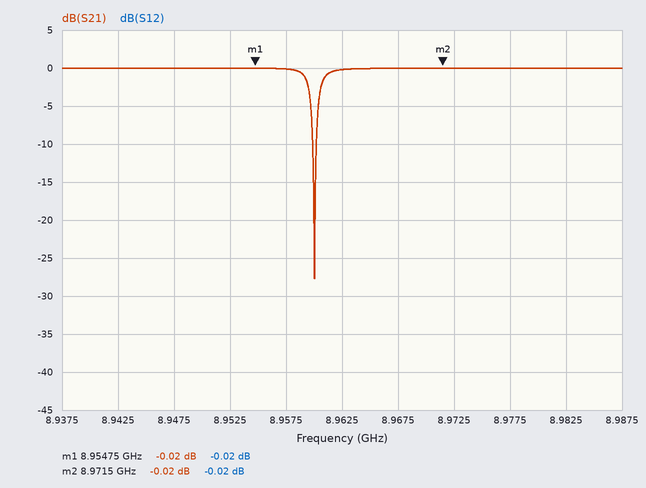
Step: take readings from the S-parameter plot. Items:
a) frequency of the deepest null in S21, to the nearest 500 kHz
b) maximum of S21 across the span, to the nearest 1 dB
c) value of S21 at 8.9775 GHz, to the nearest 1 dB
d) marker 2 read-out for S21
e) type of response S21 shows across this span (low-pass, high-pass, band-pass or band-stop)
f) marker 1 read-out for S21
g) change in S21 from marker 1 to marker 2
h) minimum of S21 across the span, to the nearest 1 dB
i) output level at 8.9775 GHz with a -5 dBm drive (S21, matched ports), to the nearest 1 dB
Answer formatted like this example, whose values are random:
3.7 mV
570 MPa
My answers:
8.9600 GHz
0 dB
0 dB
-0.02 dB
band-stop
-0.02 dB
0.00 dB
-28 dB
-5 dBm
